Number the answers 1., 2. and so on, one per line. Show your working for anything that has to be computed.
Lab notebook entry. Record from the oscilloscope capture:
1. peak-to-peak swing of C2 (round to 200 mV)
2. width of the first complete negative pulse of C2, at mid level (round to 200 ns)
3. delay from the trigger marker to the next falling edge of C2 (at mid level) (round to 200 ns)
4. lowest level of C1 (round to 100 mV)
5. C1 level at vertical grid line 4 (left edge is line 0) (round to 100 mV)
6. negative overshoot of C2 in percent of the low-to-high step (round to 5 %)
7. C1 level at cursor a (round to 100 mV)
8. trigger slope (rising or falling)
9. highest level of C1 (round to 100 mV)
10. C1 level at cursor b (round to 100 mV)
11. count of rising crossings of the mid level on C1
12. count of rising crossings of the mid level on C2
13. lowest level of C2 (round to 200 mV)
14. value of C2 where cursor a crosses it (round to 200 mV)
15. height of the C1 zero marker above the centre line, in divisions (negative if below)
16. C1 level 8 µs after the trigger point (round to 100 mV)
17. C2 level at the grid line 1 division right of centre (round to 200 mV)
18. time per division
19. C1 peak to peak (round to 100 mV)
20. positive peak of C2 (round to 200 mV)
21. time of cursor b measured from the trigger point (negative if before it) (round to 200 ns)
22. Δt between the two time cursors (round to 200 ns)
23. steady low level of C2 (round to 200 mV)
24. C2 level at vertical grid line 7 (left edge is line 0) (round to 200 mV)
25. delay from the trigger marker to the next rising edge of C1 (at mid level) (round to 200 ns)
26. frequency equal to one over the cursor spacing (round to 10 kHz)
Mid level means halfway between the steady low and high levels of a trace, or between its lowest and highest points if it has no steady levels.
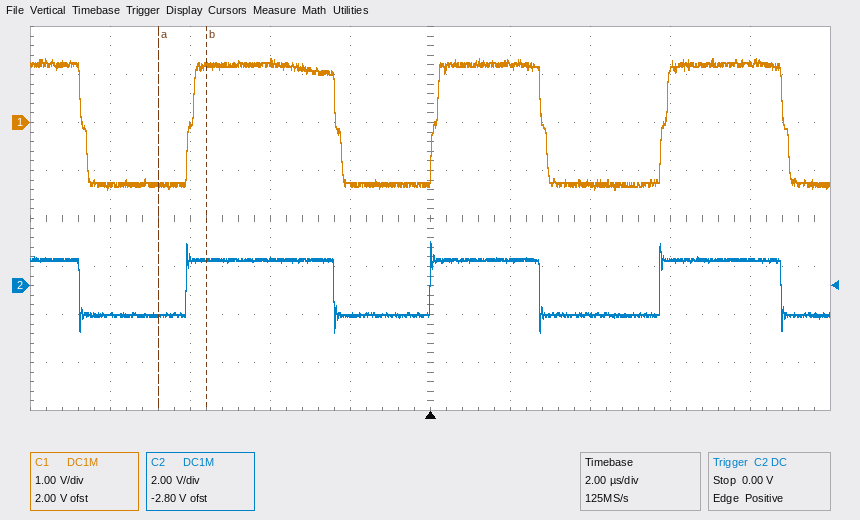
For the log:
1. 1.8 V − (-2.0 V) = 3.8 V
2. 2.6 µs
3. 2.8 µs
4. -1.4 V
5. -1.3 V
6. 30 %
7. -1.3 V
8. rising
9. 1.3 V
10. 1.2 V
11. 3
12. 3
13. -2.0 V
14. -1.2 V
15. +2.0 div
16. 1.2 V
17. 1.0 V
18. 2 µs
19. 1.3 V − (-1.4 V) = 2.7 V
20. 1.8 V
21. -5.6 µs
22. 1.2 µs
23. -1.2 V
24. -1.2 V
25. 200 ns
26. 1 / 1.2 µs ≈ 830 kHz
